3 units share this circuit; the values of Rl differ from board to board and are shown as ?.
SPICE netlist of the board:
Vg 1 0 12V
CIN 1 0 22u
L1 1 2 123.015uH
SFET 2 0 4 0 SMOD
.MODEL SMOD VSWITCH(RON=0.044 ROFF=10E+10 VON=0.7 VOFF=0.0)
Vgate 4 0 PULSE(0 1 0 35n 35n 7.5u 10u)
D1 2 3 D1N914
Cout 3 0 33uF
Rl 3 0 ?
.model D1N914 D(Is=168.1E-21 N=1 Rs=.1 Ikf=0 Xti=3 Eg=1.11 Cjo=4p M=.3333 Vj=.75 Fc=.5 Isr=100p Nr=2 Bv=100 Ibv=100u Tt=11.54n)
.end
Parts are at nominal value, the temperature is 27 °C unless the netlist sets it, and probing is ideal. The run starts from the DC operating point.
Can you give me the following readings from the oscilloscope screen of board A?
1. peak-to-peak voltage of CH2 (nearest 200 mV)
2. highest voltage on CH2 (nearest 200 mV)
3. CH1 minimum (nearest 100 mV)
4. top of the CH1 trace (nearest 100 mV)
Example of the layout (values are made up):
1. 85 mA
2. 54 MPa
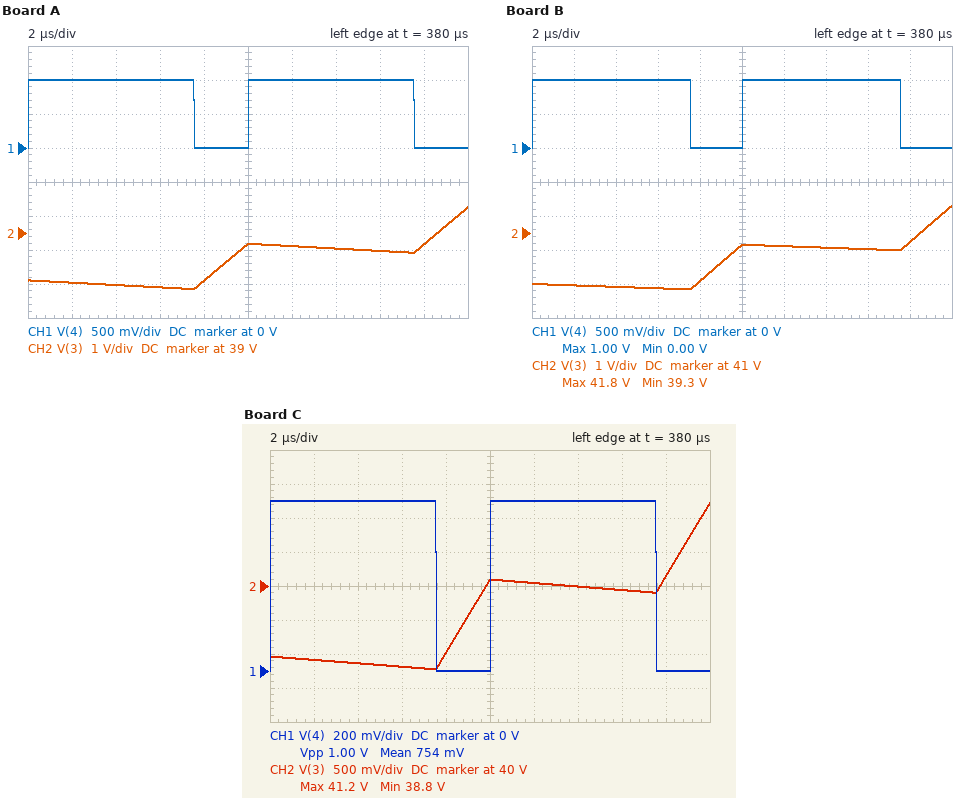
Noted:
1. 2.4 V
2. 39.8 V
3. 0 V
4. 1.0 V
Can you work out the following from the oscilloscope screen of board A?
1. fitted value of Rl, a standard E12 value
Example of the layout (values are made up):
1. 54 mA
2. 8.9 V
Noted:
1. 33 Ω
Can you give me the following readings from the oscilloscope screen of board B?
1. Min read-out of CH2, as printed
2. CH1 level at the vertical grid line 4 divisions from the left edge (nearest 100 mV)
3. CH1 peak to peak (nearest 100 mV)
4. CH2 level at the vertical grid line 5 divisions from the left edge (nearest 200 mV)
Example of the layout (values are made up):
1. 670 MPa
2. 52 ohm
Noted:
1. 39.3 V
2. 0 V
3. 1.0 V
4. 40.6 V
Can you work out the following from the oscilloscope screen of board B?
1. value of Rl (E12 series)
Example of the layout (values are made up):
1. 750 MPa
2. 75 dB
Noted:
1. 56 Ω
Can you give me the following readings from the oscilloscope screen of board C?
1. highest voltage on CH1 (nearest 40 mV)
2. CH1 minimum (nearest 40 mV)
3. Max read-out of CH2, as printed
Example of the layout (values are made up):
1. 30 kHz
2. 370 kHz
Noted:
1. 1.00 V
2. 0 V
3. 41.2 V
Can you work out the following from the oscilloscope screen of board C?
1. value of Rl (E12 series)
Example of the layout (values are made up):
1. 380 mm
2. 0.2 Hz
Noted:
1. 47 Ω
